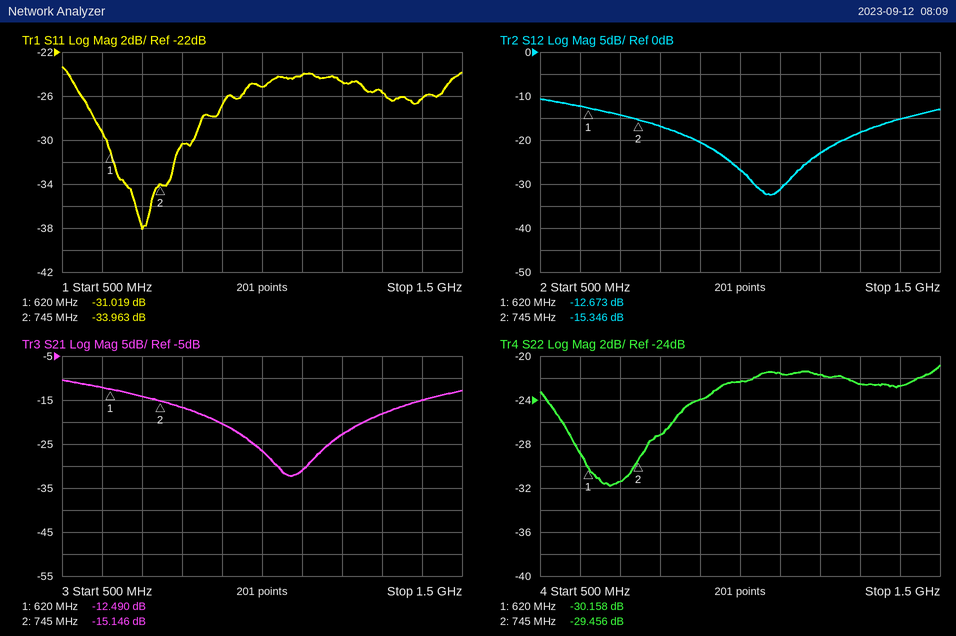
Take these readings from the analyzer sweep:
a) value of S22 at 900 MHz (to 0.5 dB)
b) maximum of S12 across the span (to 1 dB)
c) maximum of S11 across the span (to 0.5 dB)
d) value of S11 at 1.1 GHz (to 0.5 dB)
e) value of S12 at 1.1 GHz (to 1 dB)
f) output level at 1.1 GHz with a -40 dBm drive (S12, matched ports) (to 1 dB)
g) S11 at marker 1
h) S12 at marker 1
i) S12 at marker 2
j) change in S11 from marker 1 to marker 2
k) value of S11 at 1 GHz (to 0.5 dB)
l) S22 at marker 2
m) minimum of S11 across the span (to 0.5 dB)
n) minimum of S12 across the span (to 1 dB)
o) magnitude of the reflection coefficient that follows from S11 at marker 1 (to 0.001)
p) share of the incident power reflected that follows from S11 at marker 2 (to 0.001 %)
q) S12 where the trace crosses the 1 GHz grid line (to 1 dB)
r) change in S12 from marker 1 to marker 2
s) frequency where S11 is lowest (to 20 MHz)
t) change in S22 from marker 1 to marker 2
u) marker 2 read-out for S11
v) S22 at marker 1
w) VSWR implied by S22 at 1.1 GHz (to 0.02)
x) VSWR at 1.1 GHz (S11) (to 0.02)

-24.0 dB
-11 dB
-23.5 dB
-24.0 dB
-31 dB
-71 dBm
-31.019 dB
-12.673 dB
-15.346 dB
-2.944 dB
-25.0 dB
-29.456 dB
-38.0 dB
-32 dB
0.028
0.040 %
-27 dB
-2.673 dB
700 MHz
0.702 dB
-33.963 dB
-30.158 dB
1.18
1.14
